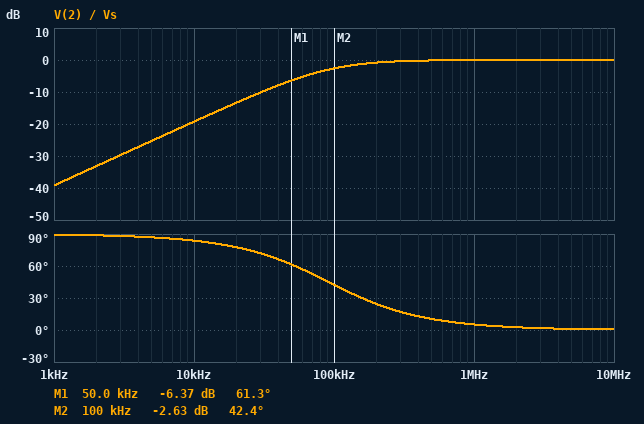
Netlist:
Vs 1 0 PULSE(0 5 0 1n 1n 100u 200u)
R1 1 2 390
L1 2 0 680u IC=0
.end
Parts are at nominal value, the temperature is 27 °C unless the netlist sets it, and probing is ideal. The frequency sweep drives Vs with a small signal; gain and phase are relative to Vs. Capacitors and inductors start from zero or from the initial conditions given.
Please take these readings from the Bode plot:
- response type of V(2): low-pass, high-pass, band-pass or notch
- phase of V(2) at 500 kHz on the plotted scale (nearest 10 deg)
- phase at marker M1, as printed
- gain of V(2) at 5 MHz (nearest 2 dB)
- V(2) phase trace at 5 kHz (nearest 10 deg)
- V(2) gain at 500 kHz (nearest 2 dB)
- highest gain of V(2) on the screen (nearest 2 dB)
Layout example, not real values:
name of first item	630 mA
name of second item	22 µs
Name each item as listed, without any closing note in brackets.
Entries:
response type of V(2): low-pass, high-pass, band-pass or notch	high-pass
phase of V(2) at 500 kHz on the plotted scale	10 deg
phase at marker M1, as printed	61.3 deg
gain of V(2) at 5 MHz	0 dB
V(2) phase trace at 5 kHz	90 deg
V(2) gain at 500 kHz	0 dB
highest gain of V(2) on the screen	0 dB
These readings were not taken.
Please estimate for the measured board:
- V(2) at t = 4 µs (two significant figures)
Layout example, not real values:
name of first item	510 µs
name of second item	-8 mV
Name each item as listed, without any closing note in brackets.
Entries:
V(2) at t = 4 µs	500 mV
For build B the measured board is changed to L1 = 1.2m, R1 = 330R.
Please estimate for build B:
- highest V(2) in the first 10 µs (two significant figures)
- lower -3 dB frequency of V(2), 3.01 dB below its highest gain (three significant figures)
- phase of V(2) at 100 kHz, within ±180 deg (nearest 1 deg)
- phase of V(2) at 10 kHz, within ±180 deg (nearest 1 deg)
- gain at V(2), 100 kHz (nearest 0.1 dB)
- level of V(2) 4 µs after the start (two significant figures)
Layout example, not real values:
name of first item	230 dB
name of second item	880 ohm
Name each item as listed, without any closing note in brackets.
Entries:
highest V(2) in the first 10 µs	5.0 V
lower -3 dB frequency of V(2), 3.01 dB below its highest gain	43.8 kHz
phase of V(2) at 100 kHz, within ±180 deg	24 deg
phase of V(2) at 10 kHz, within ±180 deg	77 deg
gain at V(2), 100 kHz	-0.8 dB
level of V(2) 4 µs after the start	1.7 V
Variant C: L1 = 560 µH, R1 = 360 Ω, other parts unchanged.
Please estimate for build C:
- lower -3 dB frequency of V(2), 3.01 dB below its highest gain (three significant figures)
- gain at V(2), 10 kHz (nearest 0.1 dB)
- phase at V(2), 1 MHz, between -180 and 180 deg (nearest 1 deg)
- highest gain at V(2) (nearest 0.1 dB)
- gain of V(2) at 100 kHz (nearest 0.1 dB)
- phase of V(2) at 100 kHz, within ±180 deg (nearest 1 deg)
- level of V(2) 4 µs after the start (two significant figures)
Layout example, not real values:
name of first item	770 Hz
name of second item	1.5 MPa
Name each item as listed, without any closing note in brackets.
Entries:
lower -3 dB frequency of V(2), 3.01 dB below its highest gain	102 kHz
gain at V(2), 10 kHz	-20.2 dB
phase at V(2), 1 MHz, between -180 and 180 deg	6 deg
highest gain at V(2)	0 dB
gain of V(2) at 100 kHz	-3.1 dB
phase of V(2) at 100 kHz, within ±180 deg	46 deg
level of V(2) 4 µs after the start	380 mV
